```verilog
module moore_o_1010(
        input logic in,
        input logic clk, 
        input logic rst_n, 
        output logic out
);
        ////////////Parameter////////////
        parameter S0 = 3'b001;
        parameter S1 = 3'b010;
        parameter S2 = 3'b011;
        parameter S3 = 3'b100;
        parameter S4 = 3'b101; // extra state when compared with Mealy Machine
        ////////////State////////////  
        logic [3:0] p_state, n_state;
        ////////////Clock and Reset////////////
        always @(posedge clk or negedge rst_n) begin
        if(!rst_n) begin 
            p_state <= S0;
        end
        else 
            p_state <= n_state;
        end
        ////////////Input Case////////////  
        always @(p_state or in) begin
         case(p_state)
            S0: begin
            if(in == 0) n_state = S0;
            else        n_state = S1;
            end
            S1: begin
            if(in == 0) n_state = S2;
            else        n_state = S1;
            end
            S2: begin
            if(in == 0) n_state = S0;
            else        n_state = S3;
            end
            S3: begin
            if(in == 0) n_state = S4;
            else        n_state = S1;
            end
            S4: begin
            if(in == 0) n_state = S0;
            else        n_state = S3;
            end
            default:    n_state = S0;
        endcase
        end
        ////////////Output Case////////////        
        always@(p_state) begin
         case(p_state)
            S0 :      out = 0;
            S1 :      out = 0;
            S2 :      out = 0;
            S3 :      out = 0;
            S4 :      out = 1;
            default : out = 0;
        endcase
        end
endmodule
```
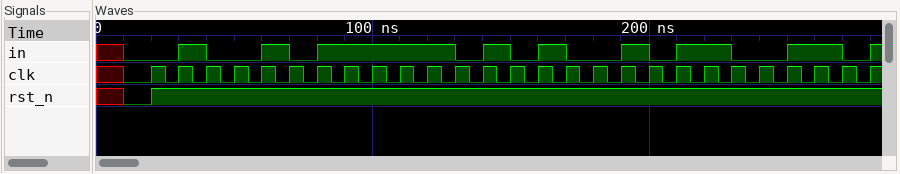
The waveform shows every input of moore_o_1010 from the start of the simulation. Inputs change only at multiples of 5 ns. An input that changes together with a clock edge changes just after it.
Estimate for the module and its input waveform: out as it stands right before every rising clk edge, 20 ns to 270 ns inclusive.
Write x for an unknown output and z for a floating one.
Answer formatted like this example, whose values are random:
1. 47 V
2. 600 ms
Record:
1. 0 0 0 0 0 0 0 0 0 0 0 0 0 0 0 1 0 1 0 0 0 0 0 0 0 0
